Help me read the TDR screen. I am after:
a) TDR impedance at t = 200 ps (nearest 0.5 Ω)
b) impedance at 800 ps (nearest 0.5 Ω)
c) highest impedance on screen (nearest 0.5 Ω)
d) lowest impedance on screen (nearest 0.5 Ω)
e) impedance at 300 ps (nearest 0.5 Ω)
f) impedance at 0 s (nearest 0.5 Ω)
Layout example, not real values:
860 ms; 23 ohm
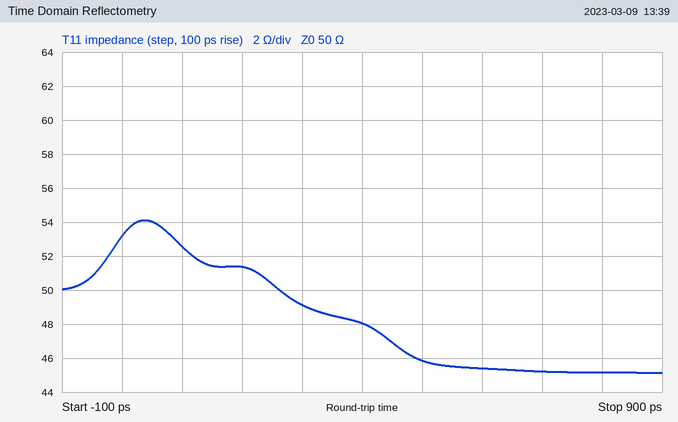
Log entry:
51.5 Ω; 45.0 Ω; 54.0 Ω; 45.0 Ω; 49.0 Ω; 53.0 Ω
